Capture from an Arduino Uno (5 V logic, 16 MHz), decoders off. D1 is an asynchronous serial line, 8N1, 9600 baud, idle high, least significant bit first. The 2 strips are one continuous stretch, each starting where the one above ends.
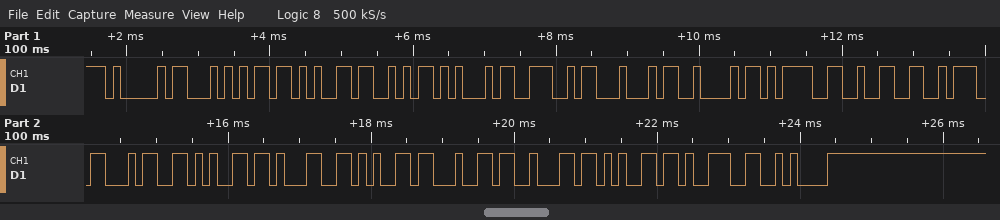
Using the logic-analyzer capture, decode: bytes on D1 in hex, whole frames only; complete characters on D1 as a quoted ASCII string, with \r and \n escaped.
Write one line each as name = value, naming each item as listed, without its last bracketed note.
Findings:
bytes on D1 in hex, whole frames only = 41 54 2B 53 45 4E 44 42 3D 32 3A 34 65 31 65 64 62 65 39 0A
complete characters on D1 as a quoted ASCII string, with \r and \n escaped = "AT+SENDB=2:4e1edbe9\n"
